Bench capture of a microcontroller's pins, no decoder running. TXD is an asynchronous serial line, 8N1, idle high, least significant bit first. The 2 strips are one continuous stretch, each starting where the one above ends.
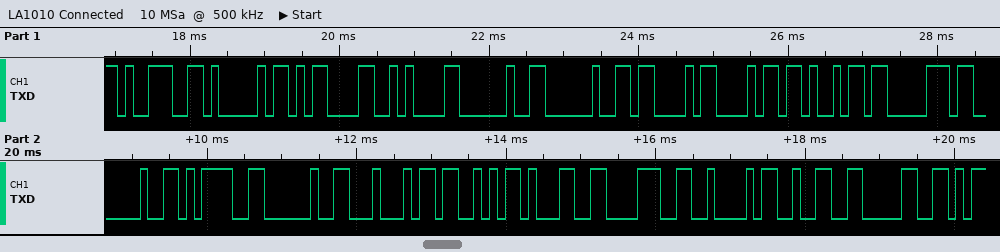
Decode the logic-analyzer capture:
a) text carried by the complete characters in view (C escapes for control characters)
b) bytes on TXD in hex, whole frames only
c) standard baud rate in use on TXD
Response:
"9A\r\n  Chip = DS18B20"
0x39 0x41 0x0D 0x0A 0x20 0x20 0x43 0x68 0x69 0x70 0x20 0x3D 0x20 0x44 0x53 0x31 0x38 0x42 0x32 0x30
9600 baud
